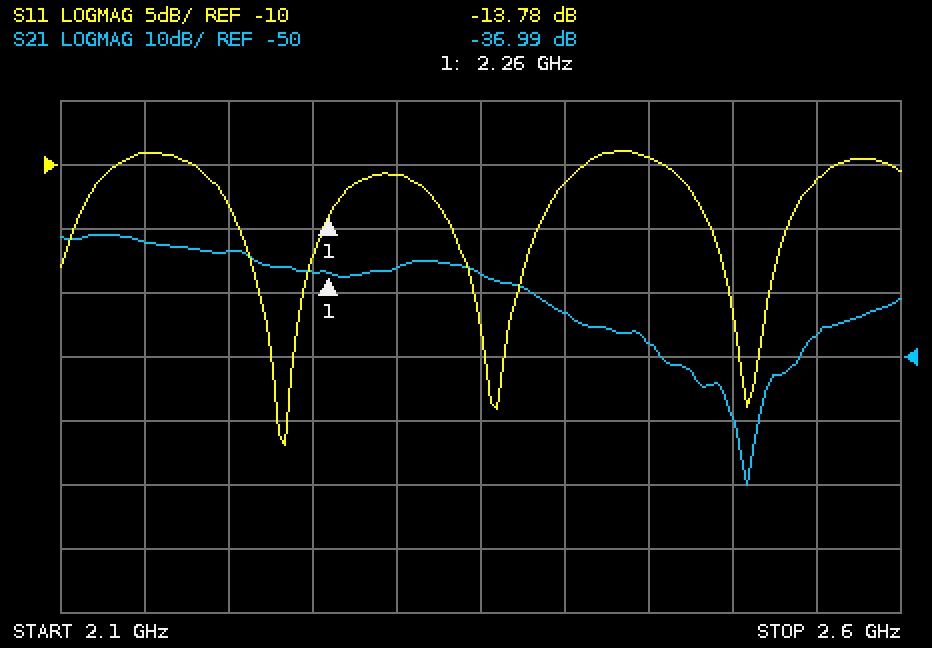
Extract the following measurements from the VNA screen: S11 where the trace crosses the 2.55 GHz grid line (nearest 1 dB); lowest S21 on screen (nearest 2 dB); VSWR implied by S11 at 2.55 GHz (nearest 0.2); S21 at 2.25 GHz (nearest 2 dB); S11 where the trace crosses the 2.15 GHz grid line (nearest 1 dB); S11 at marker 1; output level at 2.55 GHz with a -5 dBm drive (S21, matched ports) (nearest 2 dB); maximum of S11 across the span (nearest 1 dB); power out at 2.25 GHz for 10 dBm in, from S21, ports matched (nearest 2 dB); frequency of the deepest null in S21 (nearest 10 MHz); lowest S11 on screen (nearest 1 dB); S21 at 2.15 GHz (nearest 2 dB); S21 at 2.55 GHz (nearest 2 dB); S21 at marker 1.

-11 dB
-70 dB
1.8
-36 dB
-9 dB
-13.78 dB
-52 dBm
-9 dB
-26 dBm
2.51 GHz
-32 dB
-32 dB
-46 dB
-36.99 dB
